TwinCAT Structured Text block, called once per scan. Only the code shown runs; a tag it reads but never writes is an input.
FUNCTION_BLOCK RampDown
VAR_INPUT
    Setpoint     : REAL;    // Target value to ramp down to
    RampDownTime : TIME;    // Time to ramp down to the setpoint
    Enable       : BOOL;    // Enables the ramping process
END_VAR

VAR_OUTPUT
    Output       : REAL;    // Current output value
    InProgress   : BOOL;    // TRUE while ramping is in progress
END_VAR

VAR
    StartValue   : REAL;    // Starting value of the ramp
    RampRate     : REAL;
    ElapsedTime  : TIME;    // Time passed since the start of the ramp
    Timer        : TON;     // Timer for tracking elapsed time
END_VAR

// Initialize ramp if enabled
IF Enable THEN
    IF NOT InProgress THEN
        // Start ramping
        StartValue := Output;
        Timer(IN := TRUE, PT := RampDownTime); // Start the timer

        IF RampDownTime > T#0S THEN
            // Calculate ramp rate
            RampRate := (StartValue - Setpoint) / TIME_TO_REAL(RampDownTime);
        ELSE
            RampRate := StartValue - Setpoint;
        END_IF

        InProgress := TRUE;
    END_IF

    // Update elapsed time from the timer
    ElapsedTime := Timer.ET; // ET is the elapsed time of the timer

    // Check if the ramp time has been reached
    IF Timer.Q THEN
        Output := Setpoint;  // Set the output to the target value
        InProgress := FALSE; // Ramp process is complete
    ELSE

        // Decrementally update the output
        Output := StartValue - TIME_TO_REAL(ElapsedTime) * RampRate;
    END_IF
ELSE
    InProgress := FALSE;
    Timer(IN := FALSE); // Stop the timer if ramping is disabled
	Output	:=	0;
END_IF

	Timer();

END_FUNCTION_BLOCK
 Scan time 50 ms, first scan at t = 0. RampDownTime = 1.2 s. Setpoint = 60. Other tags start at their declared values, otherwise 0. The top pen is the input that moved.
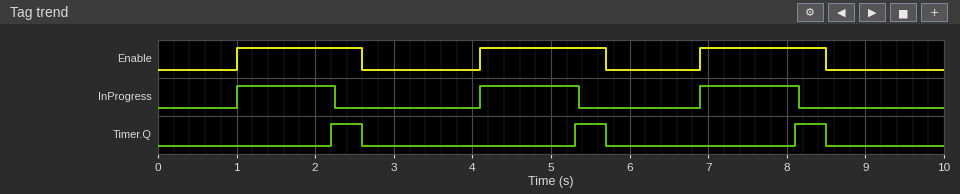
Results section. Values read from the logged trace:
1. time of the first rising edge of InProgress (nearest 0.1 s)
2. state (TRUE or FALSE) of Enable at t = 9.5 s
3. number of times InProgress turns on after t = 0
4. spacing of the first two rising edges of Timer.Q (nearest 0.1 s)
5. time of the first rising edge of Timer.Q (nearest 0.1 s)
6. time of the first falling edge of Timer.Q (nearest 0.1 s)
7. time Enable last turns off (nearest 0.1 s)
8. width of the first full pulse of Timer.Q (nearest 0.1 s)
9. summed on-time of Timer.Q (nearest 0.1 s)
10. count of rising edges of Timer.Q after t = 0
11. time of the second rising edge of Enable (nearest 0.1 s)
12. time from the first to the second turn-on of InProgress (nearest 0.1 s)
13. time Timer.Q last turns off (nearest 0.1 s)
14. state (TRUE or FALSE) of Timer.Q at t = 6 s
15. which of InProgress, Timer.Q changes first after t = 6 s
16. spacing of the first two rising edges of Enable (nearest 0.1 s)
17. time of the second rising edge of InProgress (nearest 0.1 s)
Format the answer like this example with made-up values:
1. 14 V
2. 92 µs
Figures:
1. 1.0 s
2. FALSE
3. 3
4. 3.1 s
5. 2.2 s
6. 2.6 s
7. 8.5 s
8. 0.4 s
9. 1.2 s
10. 3
11. 4.1 s
12. 3.1 s
13. 8.5 s
14. FALSE
15. InProgress
16. 3.1 s
17. 4.1 s
